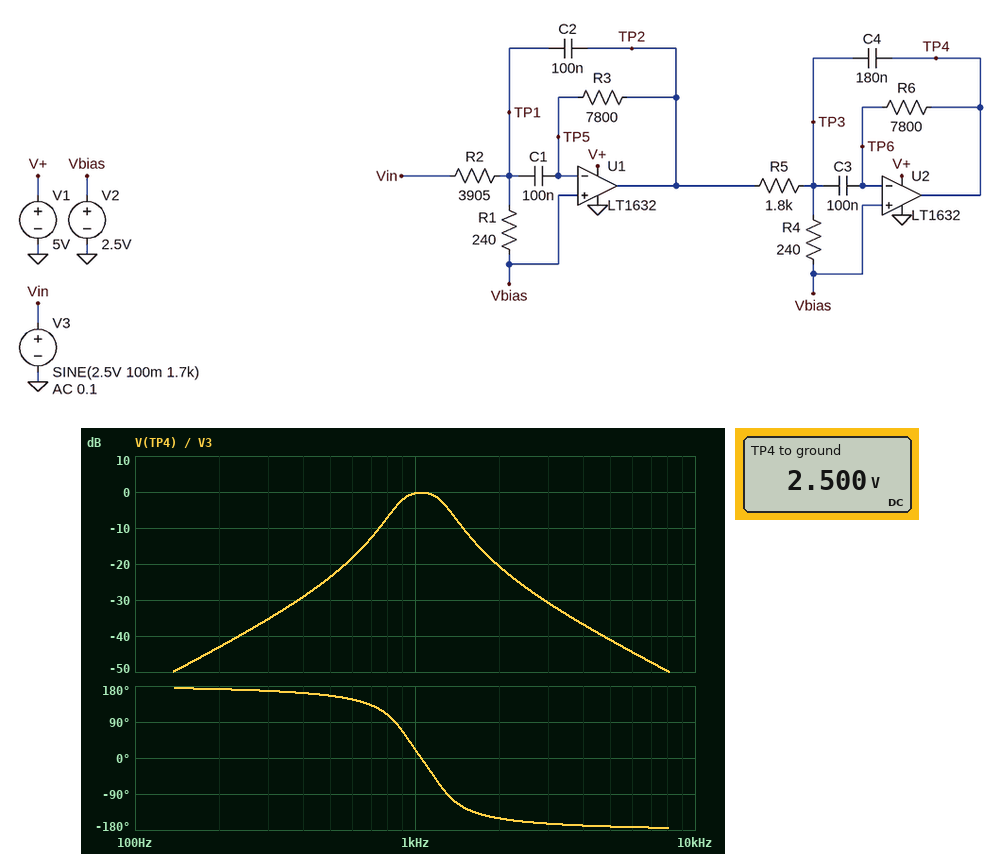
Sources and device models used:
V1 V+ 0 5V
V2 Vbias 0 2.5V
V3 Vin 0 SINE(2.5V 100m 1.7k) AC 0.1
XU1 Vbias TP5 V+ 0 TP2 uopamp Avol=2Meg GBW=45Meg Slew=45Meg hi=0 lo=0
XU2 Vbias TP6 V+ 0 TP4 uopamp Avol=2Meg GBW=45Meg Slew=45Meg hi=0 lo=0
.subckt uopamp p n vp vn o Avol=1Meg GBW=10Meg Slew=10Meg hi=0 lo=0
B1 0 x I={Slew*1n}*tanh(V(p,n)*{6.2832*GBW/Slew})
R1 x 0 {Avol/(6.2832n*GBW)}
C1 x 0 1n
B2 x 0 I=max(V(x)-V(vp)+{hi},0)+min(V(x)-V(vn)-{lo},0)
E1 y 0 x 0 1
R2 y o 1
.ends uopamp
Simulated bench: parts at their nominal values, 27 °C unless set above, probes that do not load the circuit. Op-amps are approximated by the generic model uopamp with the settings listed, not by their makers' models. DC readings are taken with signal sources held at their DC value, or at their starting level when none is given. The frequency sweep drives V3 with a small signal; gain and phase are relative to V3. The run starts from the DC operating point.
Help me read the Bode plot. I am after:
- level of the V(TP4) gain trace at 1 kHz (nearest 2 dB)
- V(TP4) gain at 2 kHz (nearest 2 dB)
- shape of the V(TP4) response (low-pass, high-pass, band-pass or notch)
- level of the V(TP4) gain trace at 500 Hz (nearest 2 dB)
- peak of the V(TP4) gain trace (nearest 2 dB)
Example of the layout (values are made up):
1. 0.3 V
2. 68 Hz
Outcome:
1. 0 dB
2. -20 dB
3. band-pass
4. -24 dB
5. 0 dB
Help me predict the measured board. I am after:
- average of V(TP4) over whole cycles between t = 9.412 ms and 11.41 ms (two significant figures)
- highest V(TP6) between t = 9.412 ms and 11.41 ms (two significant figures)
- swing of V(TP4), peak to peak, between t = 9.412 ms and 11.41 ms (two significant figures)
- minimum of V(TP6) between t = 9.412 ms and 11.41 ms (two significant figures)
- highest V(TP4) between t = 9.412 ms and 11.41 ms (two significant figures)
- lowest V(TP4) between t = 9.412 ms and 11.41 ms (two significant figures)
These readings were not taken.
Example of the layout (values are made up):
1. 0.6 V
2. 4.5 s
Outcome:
1. 2.5 V
2. 2.5 V
3. 34 mV
4. 2.5 V
5. 2.5 V
6. 2.5 V
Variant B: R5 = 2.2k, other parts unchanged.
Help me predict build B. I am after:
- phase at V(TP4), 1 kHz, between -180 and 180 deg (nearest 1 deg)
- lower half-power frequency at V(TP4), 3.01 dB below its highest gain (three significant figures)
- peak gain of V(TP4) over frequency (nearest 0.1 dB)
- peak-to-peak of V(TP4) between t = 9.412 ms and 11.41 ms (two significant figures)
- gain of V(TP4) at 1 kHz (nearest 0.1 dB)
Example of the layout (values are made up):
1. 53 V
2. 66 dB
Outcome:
1. 19 deg
2. 864 Hz
3. -2.2 dB
4. 28 mV
5. -2.3 dB
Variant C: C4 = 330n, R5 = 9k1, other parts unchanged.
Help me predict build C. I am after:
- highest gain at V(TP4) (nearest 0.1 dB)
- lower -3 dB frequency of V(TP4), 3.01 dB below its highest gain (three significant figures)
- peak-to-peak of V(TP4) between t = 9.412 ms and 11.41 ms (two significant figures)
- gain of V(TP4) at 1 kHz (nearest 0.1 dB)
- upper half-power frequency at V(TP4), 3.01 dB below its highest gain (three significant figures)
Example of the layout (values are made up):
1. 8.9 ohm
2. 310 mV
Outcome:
1. -24.1 dB
2. 613 Hz
3. 3.1 mV
4. -24.9 dB
5. 1.32 kHz
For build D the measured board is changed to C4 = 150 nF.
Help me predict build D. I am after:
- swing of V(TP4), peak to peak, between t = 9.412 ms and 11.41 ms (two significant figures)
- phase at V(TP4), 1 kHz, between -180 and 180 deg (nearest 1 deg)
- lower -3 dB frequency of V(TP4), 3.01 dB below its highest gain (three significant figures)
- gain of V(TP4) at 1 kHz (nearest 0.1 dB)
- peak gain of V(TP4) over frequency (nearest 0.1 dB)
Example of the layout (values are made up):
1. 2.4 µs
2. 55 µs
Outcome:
1. 44 mV
2. 51 deg
3. 955 Hz
4. 1.4 dB
5. 2.8 dB
